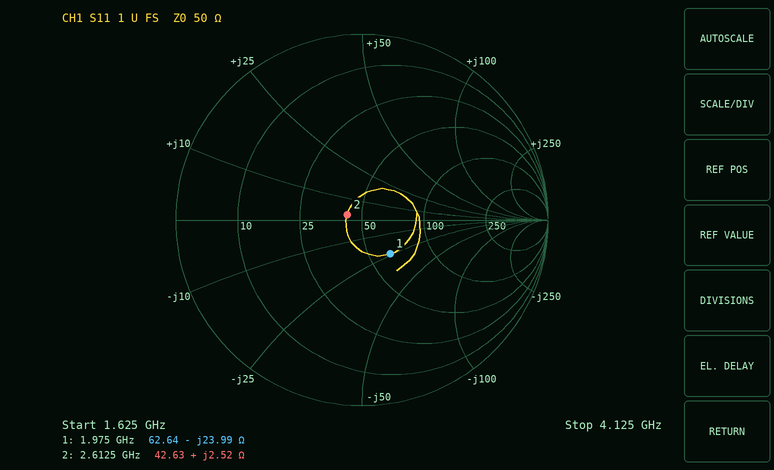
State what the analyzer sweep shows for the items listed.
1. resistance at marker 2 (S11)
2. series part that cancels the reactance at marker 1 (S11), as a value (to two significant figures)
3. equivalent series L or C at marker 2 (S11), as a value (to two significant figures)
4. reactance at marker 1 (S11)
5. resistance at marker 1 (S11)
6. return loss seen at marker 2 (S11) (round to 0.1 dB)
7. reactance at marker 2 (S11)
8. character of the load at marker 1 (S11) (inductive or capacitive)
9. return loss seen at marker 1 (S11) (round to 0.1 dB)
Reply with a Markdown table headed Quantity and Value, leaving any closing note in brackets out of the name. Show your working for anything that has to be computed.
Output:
| Quantity | Value |
|---|---|
| resistance at marker 2 | 42.63 Ω |
| series part that cancels the reactance at marker 1 (S11), as a value | L = 23.99 Ω/(2π × 1.975 GHz) ≈ 1.9 nH |
| equivalent series L or C at marker 2 (S11), as a value | L = 2.52 Ω/(2π × 2.6125 GHz) ≈ 154 pH, so 150 pH to two significant figures |
| reactance at marker 1 | -23.99 Ω |
| resistance at marker 1 | 62.64 Ω |
| return loss seen at marker 2 (S11) | 21.5 dB |
| reactance at marker 2 | +2.52 Ω |
| character of the load at marker 1 (S11) | capacitive |
| return loss seen at marker 1 (S11) | 12.6 dB |
